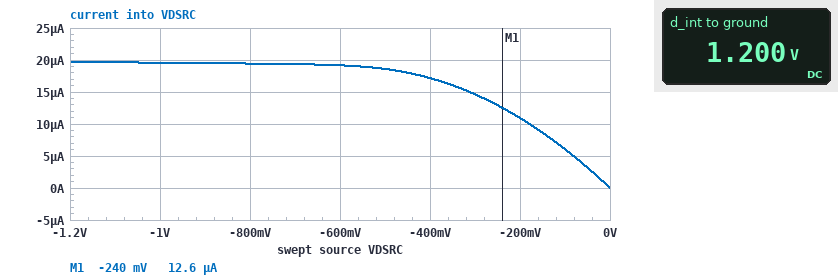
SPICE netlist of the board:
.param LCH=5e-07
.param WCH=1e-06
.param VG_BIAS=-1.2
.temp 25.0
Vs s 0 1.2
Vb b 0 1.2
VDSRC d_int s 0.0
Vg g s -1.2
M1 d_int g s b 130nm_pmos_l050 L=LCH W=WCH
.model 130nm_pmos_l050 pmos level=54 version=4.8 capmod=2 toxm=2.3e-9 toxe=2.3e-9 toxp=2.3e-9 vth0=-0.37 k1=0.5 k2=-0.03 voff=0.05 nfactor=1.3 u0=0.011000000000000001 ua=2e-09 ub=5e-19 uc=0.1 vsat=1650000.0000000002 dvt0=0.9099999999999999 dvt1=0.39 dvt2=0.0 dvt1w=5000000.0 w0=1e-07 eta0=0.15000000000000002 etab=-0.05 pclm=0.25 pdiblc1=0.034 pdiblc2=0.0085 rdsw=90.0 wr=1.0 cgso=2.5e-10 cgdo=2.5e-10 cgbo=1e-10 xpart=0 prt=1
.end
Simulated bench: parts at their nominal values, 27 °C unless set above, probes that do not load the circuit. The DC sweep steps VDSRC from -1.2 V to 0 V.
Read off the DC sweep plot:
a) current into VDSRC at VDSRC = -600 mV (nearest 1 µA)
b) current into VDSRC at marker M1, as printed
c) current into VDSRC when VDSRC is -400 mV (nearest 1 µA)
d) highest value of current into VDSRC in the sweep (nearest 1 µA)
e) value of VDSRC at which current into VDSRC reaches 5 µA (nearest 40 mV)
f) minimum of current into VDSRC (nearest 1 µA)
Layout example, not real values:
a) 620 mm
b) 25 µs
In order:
a) 19 µA
b) 12.6 µA
c) 17 µA
d) 20 µA
e) -80 mV
f) 0 A
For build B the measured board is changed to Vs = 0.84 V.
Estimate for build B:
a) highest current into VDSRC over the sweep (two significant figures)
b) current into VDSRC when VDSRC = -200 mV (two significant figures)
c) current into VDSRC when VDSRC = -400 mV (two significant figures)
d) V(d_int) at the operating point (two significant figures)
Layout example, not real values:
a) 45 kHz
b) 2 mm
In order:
a) 420 µA
b) 240 µA
c) 370 µA
d) 840 mV
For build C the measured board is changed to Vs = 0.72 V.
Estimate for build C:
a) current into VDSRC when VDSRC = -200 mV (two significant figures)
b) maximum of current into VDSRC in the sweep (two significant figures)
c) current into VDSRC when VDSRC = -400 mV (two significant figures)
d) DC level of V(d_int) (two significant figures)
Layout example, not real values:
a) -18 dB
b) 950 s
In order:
a) 230 µA
b) 390 µA
c) 350 µA
d) 720 mV
